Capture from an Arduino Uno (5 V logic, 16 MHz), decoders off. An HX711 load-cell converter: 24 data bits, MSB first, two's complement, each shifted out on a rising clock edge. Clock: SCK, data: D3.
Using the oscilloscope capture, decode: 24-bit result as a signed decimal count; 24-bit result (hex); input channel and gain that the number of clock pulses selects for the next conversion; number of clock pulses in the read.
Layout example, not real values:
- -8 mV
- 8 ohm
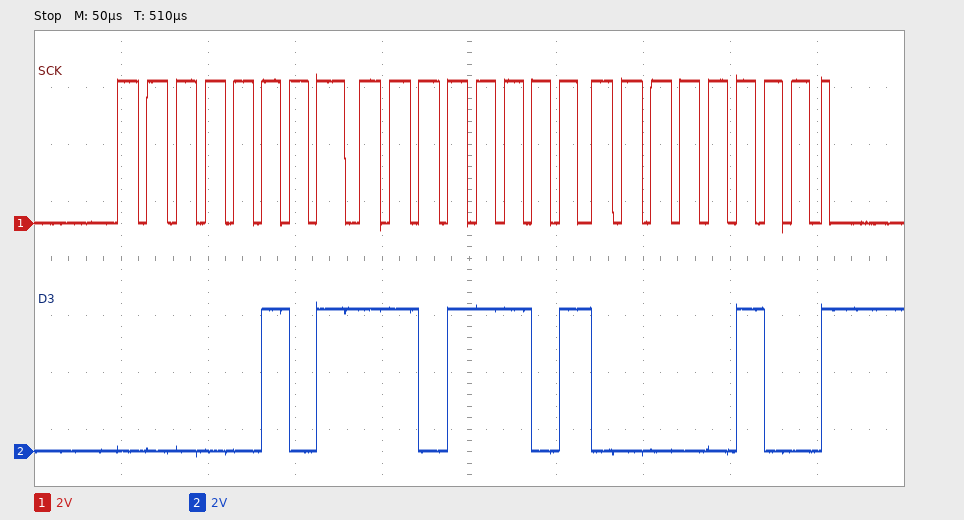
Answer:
- 384260
- 0x05DD04
- channel A, gain 128
- 25
